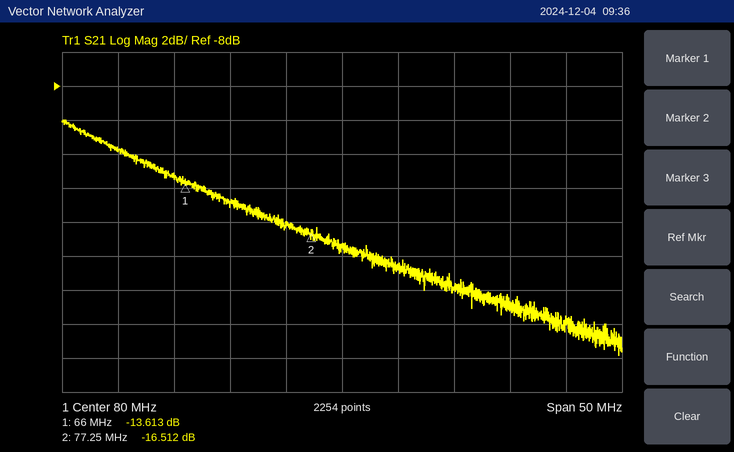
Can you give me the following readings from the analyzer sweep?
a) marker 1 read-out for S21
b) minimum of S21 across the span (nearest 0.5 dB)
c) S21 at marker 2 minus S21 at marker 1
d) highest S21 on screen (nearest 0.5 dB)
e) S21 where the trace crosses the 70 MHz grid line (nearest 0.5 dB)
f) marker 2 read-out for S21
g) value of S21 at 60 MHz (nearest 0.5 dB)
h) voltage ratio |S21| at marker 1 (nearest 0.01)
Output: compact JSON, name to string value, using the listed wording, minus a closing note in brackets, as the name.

{"marker 1 read-out for S21": "-13.613 dB", "minimum of S21 across the span": "-24.0 dB", "S21 at marker 2 minus S21 at marker 1": "-2.899 dB", "highest S21 on screen": "-10.0 dB", "S21 where the trace crosses the 70 MHz grid line": "-15.0 dB", "marker 2 read-out for S21": "-16.512 dB", "value of S21 at 60 MHz": "-12.0 dB", "voltage ratio |S21| at marker 1": "0.21"}
